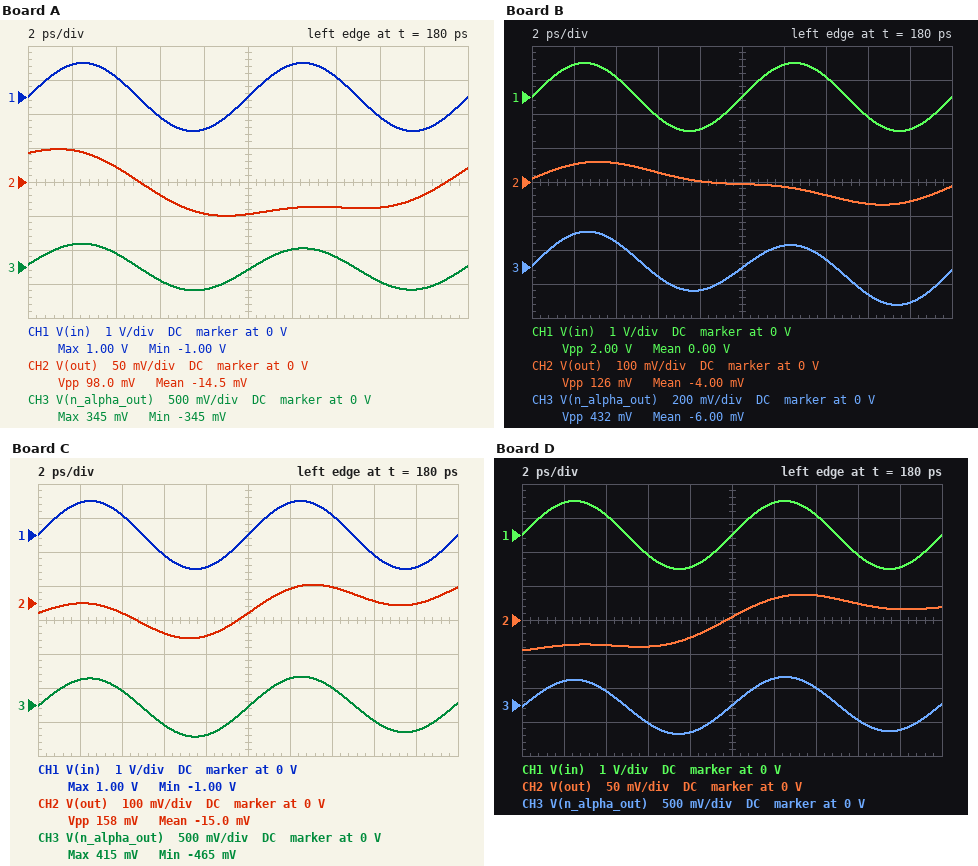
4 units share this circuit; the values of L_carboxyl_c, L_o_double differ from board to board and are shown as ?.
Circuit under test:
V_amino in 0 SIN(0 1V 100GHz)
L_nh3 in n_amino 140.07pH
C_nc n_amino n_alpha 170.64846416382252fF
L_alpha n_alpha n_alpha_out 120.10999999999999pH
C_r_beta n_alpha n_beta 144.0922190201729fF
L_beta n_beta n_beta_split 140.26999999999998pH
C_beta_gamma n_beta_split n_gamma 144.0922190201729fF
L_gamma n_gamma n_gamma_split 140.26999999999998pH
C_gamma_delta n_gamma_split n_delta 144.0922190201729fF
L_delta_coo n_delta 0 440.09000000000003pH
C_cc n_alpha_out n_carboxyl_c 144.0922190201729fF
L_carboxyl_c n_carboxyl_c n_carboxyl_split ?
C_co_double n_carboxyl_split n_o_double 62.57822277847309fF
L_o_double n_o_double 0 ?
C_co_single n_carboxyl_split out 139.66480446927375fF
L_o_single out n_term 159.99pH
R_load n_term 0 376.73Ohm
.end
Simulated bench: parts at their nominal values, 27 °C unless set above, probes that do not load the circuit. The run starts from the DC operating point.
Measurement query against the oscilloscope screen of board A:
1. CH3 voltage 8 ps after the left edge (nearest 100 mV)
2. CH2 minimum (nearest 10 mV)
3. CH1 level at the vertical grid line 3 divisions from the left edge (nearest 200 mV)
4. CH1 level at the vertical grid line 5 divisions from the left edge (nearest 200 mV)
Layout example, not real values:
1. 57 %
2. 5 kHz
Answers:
1. -300 mV
2. -50 mV
3. -600 mV
4. 0 V
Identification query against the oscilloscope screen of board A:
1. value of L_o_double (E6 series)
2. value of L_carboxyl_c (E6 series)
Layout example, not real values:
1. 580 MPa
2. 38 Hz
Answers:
1. 47 pH
2. 150 pH
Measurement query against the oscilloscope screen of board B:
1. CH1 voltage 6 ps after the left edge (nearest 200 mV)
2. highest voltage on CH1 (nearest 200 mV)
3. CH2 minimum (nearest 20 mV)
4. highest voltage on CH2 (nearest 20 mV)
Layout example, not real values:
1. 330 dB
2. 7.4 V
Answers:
1. -600 mV
2. 1.0 V
3. -60 mV
4. 60 mV
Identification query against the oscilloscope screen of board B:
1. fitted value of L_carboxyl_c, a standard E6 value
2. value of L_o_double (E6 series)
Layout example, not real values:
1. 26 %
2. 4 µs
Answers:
1. 68 pH
2. 47 pH
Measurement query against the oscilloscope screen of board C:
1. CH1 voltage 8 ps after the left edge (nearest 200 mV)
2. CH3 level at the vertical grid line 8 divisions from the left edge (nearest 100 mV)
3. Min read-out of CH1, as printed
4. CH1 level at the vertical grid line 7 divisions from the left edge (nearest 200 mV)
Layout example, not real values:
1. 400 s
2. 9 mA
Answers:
1. -1.0 V
2. -200 mV
3. -1.00 V
4. 600 mV
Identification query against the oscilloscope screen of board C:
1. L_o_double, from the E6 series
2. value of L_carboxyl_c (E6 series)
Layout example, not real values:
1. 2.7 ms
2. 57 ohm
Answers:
1. 68 pH
2. 220 pH
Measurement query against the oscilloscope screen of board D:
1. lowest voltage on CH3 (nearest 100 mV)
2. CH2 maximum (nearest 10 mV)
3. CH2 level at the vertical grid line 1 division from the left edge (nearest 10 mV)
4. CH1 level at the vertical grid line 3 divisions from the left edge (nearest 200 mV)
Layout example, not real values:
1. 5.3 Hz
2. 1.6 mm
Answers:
1. -400 mV
2. 40 mV
3. -40 mV
4. -600 mV
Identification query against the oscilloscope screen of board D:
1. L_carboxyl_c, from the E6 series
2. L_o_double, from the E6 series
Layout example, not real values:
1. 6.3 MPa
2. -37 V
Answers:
1. 220 pH
2. 47 pH
